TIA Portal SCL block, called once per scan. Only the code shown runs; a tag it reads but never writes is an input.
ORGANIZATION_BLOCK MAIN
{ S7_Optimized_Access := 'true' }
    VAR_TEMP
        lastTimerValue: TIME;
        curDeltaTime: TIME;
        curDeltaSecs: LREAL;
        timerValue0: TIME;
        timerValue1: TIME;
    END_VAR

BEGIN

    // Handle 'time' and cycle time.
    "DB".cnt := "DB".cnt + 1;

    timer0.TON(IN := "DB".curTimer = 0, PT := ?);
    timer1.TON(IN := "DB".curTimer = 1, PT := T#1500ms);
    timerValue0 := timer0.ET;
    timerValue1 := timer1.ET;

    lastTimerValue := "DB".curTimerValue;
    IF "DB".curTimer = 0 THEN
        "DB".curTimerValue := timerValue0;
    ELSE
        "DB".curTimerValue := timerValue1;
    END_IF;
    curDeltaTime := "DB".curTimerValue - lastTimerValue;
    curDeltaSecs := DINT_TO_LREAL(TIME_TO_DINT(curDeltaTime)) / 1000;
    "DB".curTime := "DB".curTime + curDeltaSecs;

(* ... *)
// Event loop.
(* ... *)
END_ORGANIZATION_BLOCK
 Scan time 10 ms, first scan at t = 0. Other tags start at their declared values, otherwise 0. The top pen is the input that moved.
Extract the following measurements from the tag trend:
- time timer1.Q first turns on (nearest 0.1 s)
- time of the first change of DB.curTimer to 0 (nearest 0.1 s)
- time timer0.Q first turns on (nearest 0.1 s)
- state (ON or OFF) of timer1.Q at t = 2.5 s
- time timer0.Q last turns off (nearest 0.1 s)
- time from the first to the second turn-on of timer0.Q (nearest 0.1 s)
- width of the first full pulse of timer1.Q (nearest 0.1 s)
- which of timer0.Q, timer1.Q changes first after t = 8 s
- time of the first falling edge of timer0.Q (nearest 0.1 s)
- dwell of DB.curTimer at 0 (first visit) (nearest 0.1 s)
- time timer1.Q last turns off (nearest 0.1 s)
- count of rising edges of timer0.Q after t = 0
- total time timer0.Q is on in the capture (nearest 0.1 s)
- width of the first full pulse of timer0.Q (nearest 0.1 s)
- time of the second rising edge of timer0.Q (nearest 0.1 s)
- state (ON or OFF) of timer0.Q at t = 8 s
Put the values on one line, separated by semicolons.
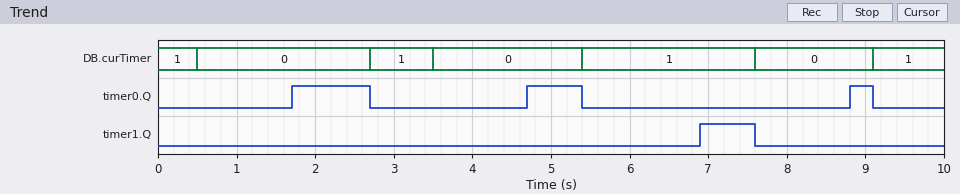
6.9 s; 0.5 s; 1.7 s; OFF; 9.1 s; 3.0 s; 0.7 s; timer0.Q; 2.7 s; 2.2 s; 7.6 s; 3; 2.0 s; 1.0 s; 4.7 s; OFF
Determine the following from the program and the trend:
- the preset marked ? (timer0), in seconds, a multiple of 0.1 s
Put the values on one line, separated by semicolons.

1.2 s
